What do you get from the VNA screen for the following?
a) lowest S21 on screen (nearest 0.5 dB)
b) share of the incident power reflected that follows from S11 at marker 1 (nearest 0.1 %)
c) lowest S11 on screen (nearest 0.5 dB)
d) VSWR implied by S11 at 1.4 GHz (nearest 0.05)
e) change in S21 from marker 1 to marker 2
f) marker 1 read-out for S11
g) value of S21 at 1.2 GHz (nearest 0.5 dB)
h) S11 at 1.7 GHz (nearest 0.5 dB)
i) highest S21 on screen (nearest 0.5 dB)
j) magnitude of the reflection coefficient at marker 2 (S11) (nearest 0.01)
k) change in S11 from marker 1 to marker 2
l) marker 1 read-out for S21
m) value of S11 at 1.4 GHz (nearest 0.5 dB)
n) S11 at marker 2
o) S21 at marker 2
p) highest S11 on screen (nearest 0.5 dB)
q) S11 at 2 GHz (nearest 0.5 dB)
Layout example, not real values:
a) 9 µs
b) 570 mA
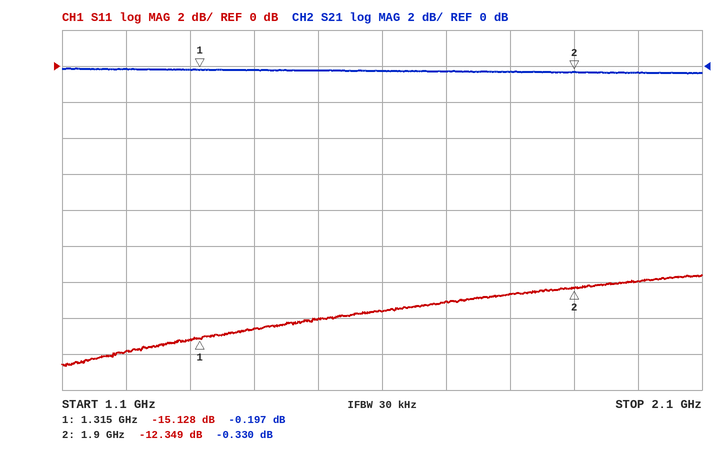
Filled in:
a) -0.5 dB
b) 3.1 %
c) -16.5 dB
d) 1.45
e) -0.133 dB
f) -15.128 dB
g) 0.0 dB
h) -13.0 dB
i) 0.0 dB
j) 0.24
k) 2.779 dB
l) -0.197 dB
m) -14.5 dB
n) -12.349 dB
o) -0.330 dB
p) -11.5 dB
q) -12.0 dB
